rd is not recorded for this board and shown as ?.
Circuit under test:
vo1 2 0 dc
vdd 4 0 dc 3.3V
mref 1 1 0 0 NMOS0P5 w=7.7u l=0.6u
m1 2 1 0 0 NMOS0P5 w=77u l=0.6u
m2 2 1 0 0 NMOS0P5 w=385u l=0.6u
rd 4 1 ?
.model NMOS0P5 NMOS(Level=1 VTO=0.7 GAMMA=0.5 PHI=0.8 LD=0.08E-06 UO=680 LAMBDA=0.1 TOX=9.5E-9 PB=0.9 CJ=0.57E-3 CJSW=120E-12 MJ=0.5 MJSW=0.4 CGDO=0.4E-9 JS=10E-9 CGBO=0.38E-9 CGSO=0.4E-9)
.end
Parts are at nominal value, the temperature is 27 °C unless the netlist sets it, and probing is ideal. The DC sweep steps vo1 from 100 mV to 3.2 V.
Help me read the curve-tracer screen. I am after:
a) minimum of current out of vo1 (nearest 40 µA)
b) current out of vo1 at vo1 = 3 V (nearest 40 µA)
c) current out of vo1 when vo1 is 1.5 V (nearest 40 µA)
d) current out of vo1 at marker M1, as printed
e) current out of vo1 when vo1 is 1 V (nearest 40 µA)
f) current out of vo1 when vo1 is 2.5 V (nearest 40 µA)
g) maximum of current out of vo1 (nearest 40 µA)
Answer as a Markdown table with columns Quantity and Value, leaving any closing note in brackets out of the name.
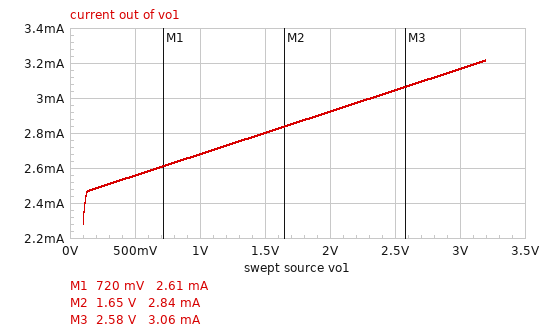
| Quantity | Value |
|---|---|
| minimum of current out of vo1 | 2.28 mA |
| current out of vo1 at vo1 = 3 V | 3.16 mA |
| current out of vo1 when vo1 is 1.5 V | 2.80 mA |
| current out of vo1 at marker M1, as printed | 2.61 mA |
| current out of vo1 when vo1 is 1 V | 2.68 mA |
| current out of vo1 when vo1 is 2.5 V | 3.04 mA |
| maximum of current out of vo1 | 3.20 mA |
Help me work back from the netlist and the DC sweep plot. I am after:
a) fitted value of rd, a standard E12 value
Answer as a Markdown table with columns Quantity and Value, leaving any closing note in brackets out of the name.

| Quantity | Value |
|---|---|
| fitted value of rd, a standard E12 value | 56 kΩ |
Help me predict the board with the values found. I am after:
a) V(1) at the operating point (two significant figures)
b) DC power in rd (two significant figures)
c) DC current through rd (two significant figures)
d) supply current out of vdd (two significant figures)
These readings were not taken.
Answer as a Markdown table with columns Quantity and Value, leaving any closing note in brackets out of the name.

| Quantity | Value |
|---|---|
| V(1) at the operating point | 840 mV |
| DC power in rd | 110 µW |
| DC current through rd | 44 µA |
| supply current out of vdd | 44 µA |
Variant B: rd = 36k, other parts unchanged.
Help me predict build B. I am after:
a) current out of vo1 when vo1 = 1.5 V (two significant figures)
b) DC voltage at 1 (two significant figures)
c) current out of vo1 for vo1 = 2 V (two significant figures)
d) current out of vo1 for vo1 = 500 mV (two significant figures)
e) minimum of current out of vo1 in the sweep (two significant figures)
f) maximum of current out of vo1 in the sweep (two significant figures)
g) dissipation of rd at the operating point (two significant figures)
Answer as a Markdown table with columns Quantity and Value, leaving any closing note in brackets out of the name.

| Quantity | Value |
|---|---|
| current out of vo1 when vo1 = 1.5 V | 4.3 mA |
| DC voltage at 1 | 870 mV |
| current out of vo1 for vo1 = 2 V | 4.5 mA |
| current out of vo1 for vo1 = 500 mV | 3.9 mA |
| minimum of current out of vo1 in the sweep | 3.1 mA |
| maximum of current out of vo1 in the sweep | 4.9 mA |
| dissipation of rd at the operating point | 160 µW |
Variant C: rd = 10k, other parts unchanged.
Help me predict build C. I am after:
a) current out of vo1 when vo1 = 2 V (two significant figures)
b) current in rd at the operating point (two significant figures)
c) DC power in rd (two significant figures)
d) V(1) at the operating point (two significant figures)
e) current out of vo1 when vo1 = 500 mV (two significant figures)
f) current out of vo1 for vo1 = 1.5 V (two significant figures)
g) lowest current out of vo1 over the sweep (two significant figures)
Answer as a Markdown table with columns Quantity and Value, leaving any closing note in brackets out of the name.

| Quantity | Value |
|---|---|
| current out of vo1 when vo1 = 2 V | 15 mA |
| current in rd at the operating point | 230 µA |
| DC power in rd | 520 µW |
| V(1) at the operating point | 1.0 V |
| current out of vo1 when vo1 = 500 mV | 13 mA |
| current out of vo1 for vo1 = 1.5 V | 14 mA |
| lowest current out of vo1 over the sweep | 6.8 mA |
